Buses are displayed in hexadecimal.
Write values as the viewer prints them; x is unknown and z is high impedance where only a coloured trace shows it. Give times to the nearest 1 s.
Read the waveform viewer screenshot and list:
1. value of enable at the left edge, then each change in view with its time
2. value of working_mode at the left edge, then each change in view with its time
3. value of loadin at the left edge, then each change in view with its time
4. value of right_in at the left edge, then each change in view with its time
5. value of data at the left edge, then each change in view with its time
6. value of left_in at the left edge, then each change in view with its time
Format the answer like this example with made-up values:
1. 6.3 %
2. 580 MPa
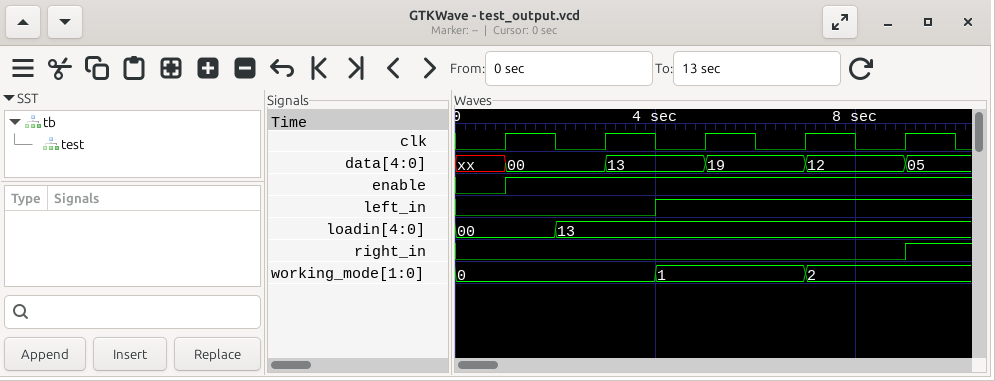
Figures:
1. 0, 1 at 1 s
2. 0, 1 at 4 s, 2 at 7 s
3. 00, 13 at 2 s
4. 0, 1 at 9 s
5. xx, 00 at 1 s, 13 at 3 s, 19 at 5 s, 12 at 7 s, 05 at 9 s
6. 0, 1 at 4 s
